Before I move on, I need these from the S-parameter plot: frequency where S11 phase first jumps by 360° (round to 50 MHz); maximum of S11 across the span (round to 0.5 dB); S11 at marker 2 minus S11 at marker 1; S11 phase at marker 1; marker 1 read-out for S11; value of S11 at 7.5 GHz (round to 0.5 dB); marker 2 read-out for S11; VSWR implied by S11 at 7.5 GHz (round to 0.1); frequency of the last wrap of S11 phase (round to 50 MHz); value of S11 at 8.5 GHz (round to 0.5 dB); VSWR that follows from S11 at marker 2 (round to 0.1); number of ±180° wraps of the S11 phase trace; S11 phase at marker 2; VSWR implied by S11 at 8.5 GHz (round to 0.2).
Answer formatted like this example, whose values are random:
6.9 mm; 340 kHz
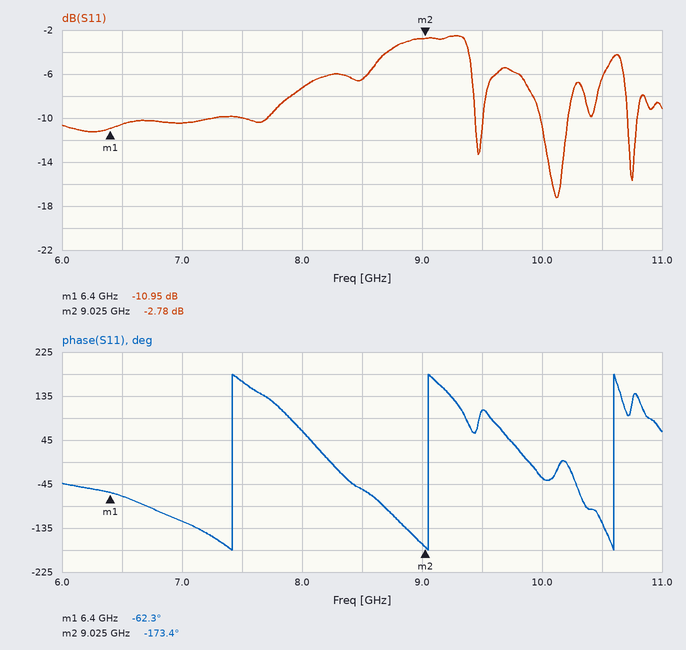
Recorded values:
7.40 GHz; -2.5 dB; 8.17 dB; -62.3°; -10.95 dB; -10.0 dB; -2.78 dB; 1.9; 10.60 GHz; -6.5 dB; 6.3; 3; -173.4°; 2.8
